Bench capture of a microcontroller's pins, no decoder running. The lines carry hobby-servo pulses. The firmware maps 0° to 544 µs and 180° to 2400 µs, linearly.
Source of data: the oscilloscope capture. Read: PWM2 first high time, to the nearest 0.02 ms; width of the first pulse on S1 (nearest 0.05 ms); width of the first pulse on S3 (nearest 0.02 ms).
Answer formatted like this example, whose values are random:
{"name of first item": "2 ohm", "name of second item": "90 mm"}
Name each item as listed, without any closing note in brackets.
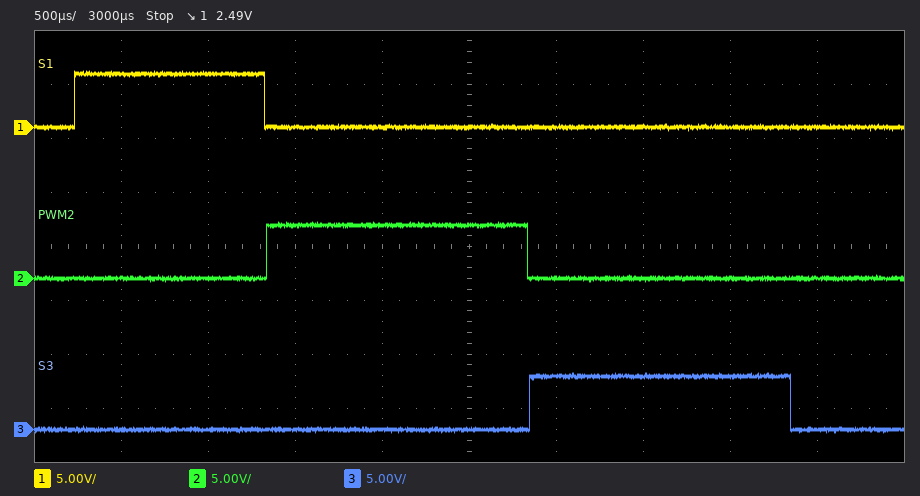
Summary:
{"PWM2 first high time, to the nearest 0.02 ms": "1.50 ms", "width of the first pulse on S1": "1.10 ms", "width of the first pulse on S3": "1.50 ms"}
